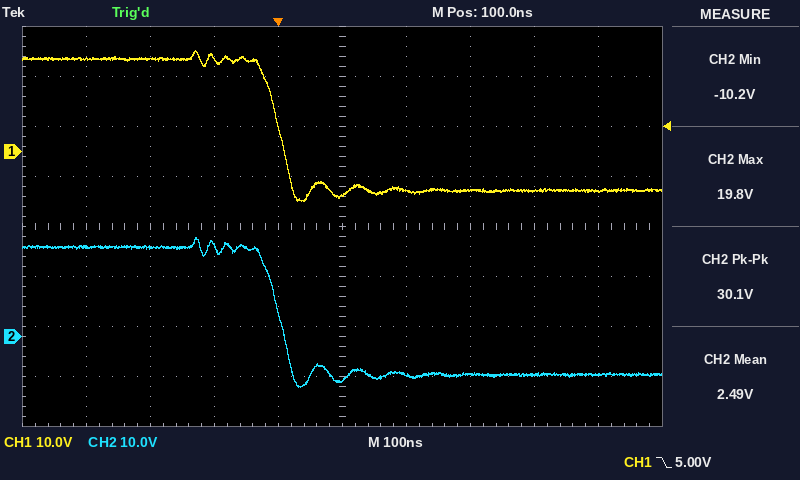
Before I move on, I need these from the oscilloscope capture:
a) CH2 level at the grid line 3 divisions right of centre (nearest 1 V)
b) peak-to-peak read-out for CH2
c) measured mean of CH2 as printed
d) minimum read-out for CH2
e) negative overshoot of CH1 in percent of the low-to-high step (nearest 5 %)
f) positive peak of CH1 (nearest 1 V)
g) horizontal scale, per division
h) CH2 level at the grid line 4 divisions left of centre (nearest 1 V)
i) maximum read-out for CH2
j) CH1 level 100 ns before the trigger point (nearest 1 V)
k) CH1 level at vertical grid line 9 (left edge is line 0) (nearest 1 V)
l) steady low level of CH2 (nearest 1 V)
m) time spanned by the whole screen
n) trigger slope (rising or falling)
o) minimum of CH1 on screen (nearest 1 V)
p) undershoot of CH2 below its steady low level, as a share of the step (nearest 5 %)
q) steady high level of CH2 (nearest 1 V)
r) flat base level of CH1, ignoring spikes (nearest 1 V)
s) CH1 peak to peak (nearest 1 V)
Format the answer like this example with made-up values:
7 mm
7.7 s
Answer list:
-8 V
30.1 V
2.49 V
-10.2 V
10 %
20 V
100 ns
18 V
19.8 V
19 V
-8 V
-8 V
1 µs
falling
-10 V
10 %
18 V
-8 V
30 V
